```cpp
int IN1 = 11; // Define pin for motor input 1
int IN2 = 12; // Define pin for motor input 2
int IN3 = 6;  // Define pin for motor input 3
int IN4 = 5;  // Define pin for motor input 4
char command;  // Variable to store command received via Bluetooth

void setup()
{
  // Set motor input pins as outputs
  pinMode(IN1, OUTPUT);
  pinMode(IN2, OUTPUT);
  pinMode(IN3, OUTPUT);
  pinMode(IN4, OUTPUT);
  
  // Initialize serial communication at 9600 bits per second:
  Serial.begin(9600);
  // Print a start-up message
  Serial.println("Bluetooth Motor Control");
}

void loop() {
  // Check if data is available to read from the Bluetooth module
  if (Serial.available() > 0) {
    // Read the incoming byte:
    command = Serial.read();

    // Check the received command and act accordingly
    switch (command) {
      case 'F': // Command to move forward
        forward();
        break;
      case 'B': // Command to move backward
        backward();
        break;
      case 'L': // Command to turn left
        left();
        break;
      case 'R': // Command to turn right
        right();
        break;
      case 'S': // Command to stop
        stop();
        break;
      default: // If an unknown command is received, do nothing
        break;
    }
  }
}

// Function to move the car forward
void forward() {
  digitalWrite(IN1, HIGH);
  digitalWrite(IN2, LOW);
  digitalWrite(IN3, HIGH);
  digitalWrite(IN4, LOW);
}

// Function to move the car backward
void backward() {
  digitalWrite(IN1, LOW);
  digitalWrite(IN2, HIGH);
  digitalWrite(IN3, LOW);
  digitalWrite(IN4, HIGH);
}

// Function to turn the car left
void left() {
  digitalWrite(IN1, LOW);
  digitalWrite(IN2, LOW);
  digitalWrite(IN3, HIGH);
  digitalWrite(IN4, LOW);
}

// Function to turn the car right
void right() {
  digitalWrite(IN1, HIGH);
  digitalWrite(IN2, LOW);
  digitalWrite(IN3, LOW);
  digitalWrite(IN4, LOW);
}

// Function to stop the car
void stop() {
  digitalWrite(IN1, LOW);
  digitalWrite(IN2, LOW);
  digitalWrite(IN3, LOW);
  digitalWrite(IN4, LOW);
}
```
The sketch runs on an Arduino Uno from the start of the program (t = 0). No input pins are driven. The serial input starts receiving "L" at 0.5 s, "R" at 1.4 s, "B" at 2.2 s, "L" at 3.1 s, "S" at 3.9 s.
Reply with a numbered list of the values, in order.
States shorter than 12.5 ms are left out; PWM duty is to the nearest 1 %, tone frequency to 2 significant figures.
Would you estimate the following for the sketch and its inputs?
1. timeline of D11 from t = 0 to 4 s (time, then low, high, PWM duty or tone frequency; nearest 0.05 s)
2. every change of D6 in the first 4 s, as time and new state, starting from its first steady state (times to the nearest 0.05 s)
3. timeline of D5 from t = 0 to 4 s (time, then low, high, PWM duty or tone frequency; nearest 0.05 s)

1. 0 s low; 1.4 s high; 2.2 s low
2. 0 s low; 0.5 s high; 1.4 s low; 3.1 s high; 3.9 s low
3. 0 s low; 2.2 s high; 3.1 s low
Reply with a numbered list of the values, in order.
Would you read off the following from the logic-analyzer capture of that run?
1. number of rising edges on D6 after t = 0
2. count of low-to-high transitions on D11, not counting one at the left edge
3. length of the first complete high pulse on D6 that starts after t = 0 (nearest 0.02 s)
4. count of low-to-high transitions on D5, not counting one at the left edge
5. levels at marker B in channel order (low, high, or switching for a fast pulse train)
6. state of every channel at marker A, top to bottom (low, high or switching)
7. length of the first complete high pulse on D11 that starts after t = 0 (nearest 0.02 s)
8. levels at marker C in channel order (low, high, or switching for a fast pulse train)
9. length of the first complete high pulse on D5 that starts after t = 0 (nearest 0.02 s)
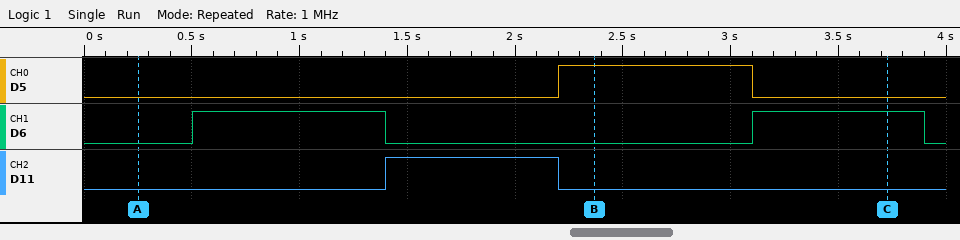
1. 2
2. 1
3. 0.90 s
4. 1
5. D5 high, D6 low, D11 low
6. D5 low, D6 low, D11 low
7. 0.80 s
8. D5 low, D6 high, D11 low
9. 0.90 s
